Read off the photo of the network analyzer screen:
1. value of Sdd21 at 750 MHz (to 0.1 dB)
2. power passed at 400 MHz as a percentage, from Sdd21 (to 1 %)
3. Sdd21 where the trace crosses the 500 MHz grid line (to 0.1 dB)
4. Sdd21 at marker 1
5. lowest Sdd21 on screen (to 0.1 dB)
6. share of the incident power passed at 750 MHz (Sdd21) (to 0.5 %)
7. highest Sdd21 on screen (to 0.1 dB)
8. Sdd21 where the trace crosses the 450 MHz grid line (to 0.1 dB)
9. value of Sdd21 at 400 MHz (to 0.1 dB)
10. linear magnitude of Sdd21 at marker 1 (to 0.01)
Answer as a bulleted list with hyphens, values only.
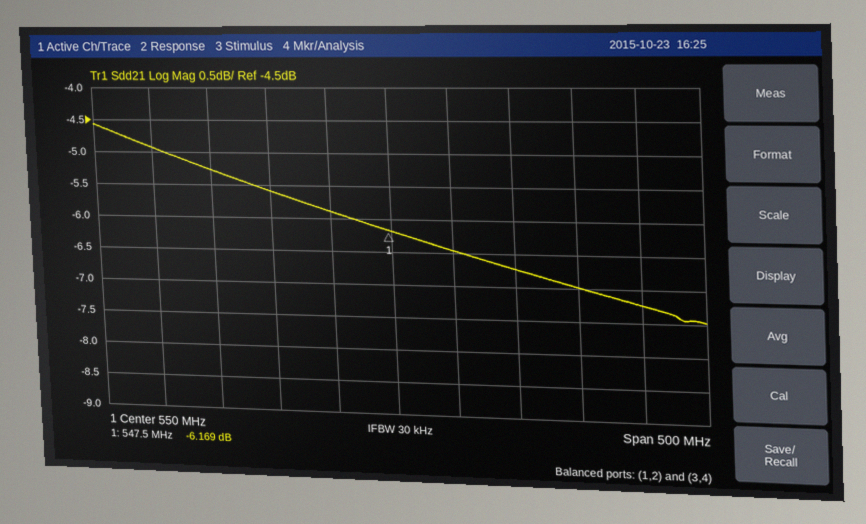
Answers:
- -7.2 dB
- 30 %
- -5.9 dB
- -6.169 dB
- -7.5 dB
- 19.0 %
- -4.6 dB
- -5.6 dB
- -5.3 dB
- 0.49
